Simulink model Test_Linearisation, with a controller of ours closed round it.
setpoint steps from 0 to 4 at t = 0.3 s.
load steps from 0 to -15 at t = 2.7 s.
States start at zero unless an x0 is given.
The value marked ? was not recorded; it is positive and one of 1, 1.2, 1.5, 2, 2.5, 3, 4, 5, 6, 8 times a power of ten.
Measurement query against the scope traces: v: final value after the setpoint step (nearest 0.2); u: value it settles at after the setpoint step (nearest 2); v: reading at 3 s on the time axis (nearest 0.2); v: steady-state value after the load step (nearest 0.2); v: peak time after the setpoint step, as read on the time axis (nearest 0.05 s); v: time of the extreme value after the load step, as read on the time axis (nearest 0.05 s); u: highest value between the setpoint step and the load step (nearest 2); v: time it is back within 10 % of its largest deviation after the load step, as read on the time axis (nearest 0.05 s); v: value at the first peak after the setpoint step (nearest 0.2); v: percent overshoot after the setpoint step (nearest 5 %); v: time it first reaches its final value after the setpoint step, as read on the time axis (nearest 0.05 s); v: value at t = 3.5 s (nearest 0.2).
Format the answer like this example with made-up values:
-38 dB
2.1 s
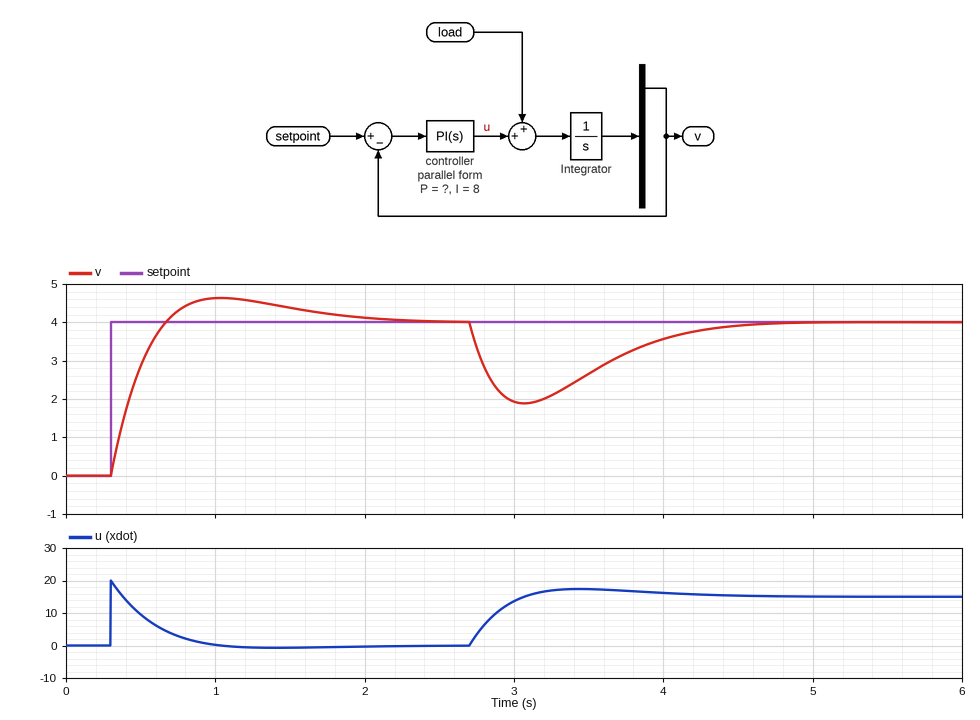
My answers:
4.0
0
2.0
4.0
1.05 s
3.05 s
20
4.25 s
4.6
15 %
0.65 s
2.6
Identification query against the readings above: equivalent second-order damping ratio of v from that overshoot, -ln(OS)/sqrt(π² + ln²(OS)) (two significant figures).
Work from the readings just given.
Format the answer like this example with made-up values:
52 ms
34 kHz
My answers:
0.52
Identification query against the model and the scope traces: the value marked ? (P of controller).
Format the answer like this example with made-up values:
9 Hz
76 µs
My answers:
5
